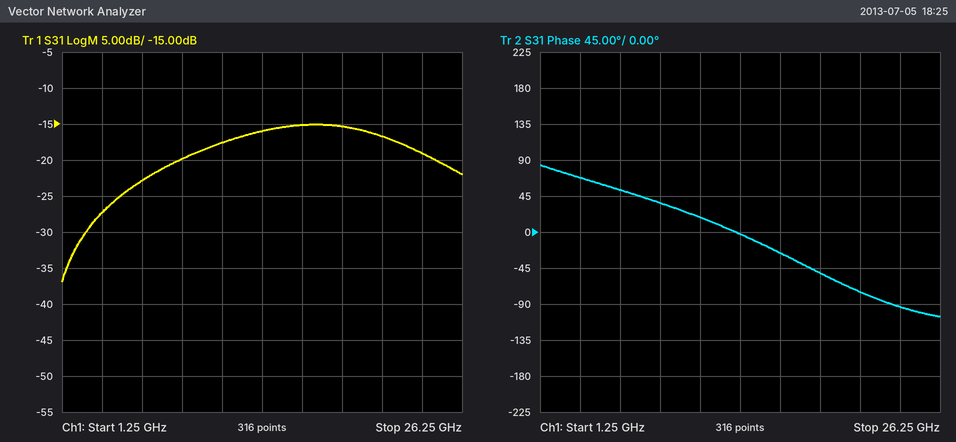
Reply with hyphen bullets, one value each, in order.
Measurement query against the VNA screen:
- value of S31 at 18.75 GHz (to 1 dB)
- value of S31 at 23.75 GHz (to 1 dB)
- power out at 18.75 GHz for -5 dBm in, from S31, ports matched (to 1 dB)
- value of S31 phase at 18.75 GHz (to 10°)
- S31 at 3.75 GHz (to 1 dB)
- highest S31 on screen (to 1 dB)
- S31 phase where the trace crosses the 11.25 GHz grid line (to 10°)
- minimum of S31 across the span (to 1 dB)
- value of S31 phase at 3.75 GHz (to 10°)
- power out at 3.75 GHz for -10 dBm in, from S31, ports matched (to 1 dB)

- -15 dB
- -19 dB
- -20 dBm
- -50°
- -27 dB
- -15 dB
- 20°
- -37 dB
- 70°
- -37 dBm
